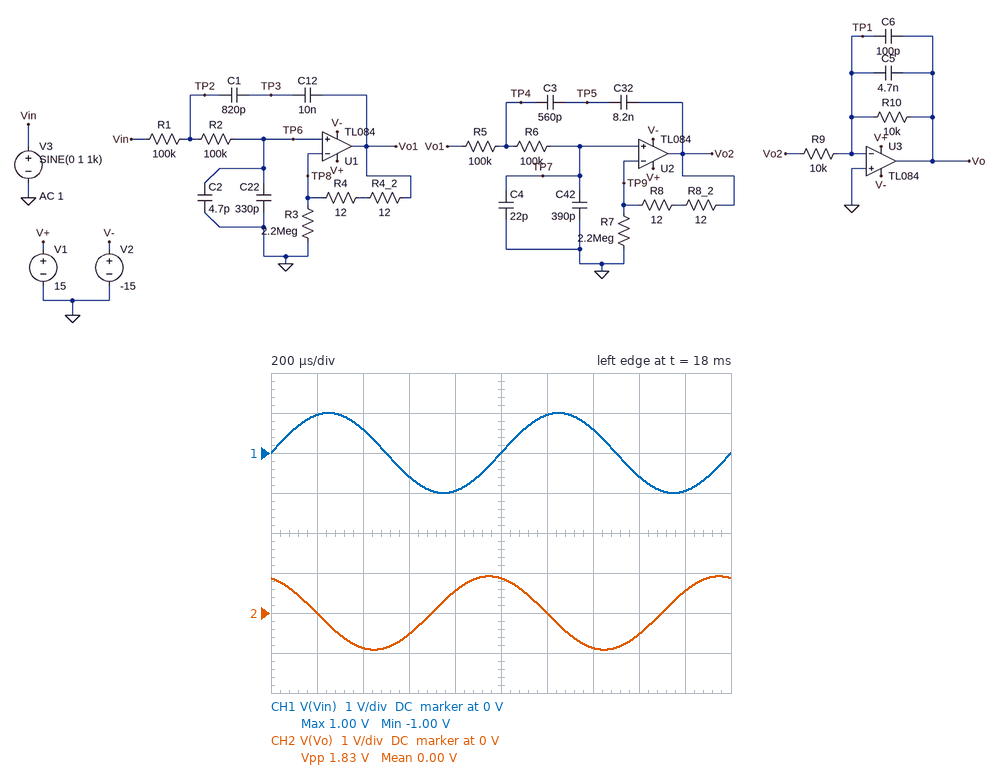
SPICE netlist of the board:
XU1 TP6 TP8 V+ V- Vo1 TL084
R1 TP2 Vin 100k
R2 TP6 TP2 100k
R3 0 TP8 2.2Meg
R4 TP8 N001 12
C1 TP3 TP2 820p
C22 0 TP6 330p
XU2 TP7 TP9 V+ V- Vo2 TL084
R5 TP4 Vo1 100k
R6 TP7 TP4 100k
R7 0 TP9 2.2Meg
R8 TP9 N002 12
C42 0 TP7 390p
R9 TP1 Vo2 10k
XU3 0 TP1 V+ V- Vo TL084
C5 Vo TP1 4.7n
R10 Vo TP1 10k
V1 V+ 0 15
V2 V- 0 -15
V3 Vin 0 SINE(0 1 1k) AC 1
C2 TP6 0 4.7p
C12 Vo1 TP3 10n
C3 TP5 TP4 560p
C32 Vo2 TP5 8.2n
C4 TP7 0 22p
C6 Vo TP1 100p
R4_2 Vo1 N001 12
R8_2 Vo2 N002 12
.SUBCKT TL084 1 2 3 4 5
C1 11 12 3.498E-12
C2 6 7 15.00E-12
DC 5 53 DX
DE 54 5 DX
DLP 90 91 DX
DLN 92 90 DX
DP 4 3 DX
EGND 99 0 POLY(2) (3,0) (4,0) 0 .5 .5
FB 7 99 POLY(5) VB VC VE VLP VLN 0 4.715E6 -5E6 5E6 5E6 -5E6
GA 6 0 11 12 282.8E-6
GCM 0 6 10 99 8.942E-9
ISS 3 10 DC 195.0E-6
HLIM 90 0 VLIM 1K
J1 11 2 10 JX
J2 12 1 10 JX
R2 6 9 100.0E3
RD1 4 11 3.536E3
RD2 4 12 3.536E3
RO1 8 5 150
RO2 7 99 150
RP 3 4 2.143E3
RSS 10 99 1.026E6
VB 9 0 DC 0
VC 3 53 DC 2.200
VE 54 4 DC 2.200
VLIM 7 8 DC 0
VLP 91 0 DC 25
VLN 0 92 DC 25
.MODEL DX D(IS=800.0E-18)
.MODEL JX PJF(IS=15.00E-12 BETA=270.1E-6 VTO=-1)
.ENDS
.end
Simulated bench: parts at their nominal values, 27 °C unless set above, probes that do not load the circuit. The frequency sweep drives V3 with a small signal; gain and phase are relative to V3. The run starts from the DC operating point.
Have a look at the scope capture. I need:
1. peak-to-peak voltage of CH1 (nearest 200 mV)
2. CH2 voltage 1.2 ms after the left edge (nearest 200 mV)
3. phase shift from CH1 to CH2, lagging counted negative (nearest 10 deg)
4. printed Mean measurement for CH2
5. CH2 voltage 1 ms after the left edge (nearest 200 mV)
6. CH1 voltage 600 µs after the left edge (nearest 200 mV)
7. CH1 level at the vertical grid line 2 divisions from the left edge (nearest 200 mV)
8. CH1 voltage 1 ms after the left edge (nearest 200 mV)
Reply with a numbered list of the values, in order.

1. 2.0 V
2. 0 V
3. 110 deg
4. 0.00 V
5. 800 mV
6. -600 mV
7. 600 mV
8. 0 V
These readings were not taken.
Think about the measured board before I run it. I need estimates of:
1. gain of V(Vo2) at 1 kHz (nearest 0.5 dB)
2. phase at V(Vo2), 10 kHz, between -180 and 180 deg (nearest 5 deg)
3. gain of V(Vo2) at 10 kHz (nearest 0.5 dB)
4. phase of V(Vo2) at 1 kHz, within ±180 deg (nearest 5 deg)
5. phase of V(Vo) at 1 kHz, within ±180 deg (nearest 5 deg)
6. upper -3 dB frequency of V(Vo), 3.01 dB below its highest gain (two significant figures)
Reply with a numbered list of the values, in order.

1. -0.5 dB
2. 60 deg
3. -39.0 dB
4. -55 deg
5. 110 deg
6. 1.9 kHz
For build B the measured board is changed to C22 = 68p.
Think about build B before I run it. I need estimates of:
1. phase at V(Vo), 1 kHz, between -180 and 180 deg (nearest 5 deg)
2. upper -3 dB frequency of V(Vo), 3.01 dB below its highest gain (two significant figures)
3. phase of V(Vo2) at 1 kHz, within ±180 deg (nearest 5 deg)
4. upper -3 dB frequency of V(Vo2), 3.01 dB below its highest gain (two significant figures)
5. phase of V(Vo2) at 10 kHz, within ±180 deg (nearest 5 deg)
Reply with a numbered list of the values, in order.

1. 130 deg
2. 2.2 kHz
3. -35 deg
4. 3.4 kHz
5. 70 deg
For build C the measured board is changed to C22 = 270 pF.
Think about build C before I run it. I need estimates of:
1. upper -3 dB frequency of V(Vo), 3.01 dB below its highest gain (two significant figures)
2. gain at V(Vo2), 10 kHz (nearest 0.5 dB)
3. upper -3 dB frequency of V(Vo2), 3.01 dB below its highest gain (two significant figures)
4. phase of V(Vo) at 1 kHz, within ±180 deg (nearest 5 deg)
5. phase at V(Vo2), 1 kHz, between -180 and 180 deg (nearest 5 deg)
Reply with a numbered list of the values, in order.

1. 2.1 kHz
2. -37.5 dB
3. 2.6 kHz
4. 115 deg
5. -50 deg
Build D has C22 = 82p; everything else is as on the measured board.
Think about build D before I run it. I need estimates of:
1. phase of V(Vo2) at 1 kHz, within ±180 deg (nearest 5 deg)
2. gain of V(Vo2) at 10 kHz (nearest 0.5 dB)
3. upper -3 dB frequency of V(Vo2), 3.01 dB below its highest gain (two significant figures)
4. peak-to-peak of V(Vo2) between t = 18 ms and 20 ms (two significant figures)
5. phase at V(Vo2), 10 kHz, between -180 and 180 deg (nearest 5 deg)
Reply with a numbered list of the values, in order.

1. -35 deg
2. -25.0 dB
3. 3.5 kHz
4. 1.9 V
5. 70 deg
